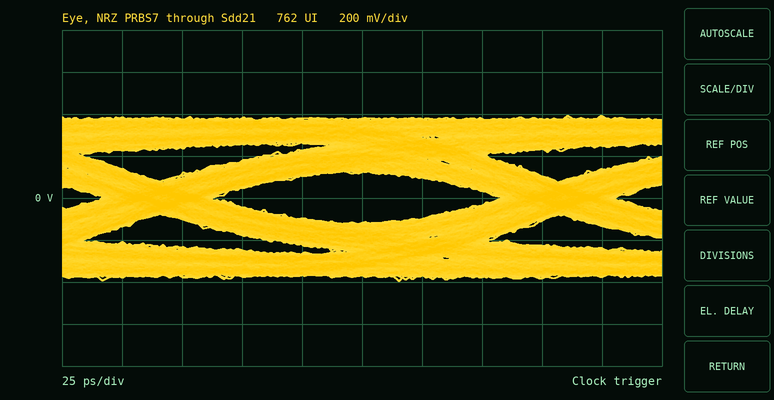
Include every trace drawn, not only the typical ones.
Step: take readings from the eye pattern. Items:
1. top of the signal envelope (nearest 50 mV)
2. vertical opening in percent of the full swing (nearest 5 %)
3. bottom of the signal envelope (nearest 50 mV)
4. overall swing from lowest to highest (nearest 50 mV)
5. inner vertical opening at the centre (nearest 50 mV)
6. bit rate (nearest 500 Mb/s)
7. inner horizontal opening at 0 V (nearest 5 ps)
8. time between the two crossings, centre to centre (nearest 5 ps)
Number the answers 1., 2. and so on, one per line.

1. 400 mV
2. 30 %
3. -400 mV
4. 800 mV
5. 250 mV
6. 6.0 Gb/s
7. 120 ps
8. 165 ps
